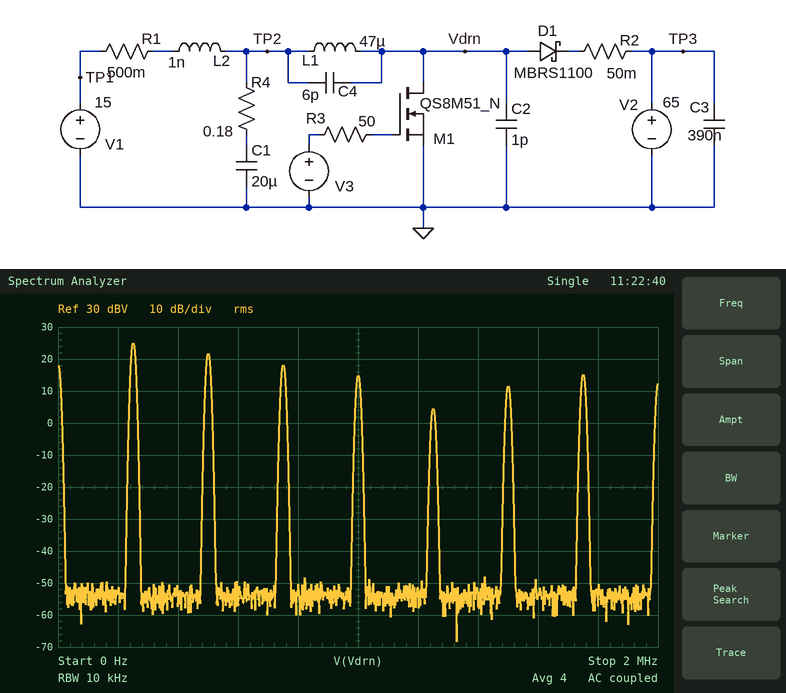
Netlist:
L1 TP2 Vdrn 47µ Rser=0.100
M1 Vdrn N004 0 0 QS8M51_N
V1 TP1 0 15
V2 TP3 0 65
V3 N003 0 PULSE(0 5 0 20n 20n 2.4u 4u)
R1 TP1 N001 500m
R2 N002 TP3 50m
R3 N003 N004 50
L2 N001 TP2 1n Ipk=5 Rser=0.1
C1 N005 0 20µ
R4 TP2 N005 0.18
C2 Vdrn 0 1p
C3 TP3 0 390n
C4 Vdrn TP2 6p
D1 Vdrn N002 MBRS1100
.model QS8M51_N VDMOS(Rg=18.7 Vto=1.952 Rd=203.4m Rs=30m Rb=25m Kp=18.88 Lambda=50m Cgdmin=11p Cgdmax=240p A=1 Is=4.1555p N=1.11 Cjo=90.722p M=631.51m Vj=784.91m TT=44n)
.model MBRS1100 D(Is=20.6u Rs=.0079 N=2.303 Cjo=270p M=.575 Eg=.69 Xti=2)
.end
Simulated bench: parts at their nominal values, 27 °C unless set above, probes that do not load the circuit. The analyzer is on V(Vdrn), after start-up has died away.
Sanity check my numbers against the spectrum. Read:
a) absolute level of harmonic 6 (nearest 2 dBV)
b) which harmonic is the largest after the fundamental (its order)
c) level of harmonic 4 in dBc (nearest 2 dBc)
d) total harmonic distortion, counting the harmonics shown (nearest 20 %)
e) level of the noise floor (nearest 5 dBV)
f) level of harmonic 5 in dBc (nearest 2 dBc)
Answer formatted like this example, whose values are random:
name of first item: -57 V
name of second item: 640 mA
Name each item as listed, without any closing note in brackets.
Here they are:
absolute level of harmonic 6: 12 dBV
which harmonic is the largest after the fundamental: 2
level of harmonic 4 in dBc: -10 dBc
total harmonic distortion, counting the harmonics shown: 100 %
level of the noise floor: -55 dBV
level of harmonic 5 in dBc: -20 dBc
